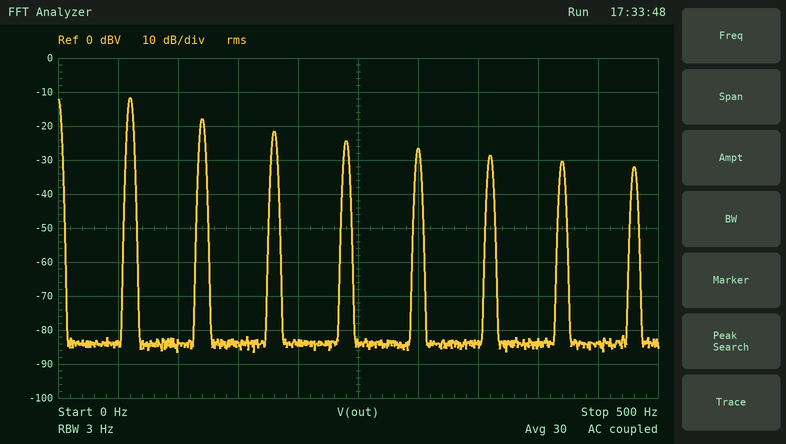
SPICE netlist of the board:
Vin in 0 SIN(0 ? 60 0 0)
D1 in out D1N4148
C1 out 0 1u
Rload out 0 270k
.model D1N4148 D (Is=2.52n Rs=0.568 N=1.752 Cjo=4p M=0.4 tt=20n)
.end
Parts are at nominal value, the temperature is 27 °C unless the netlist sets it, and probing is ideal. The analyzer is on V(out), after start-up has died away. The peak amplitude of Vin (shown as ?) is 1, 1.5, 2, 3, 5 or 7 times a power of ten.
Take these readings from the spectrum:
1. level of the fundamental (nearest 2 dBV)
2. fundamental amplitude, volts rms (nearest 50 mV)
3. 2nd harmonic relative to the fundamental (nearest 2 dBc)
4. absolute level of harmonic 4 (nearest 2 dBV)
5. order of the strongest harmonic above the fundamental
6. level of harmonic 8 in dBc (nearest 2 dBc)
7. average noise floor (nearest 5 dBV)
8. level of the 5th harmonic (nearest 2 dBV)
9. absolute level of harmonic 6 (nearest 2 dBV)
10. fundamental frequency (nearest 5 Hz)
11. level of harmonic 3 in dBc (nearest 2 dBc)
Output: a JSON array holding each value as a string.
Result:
["-12 dBV", "250 mV", "-6 dBc", "-24 dBV", "2", "-20 dBc", "-85 dBV", "-26 dBV", "-28 dBV", "60 Hz", "-10 dBc"]
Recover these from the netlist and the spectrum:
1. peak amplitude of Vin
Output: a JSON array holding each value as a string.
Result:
["20 V"]
